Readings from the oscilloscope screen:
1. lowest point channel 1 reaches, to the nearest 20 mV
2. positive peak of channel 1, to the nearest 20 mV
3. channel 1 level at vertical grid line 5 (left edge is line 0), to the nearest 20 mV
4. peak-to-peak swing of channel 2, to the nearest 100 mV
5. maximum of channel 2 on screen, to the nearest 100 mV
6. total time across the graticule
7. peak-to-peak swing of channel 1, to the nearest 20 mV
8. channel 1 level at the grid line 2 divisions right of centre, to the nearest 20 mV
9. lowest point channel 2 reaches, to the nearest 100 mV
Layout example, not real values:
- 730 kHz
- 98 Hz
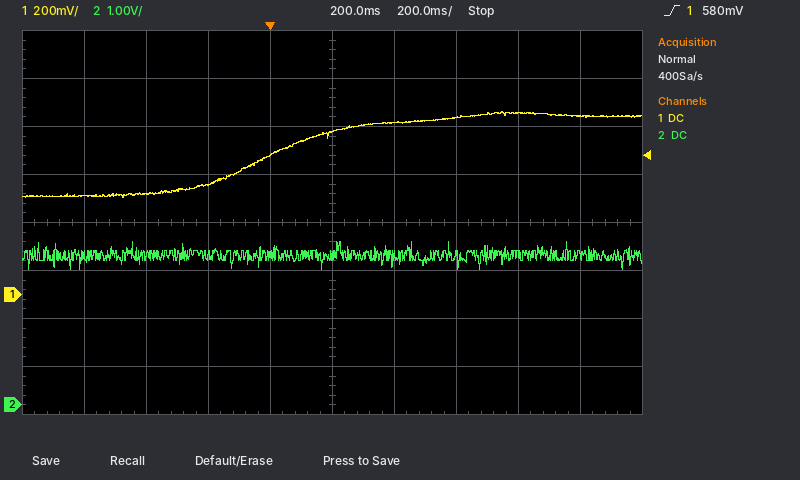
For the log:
- 400 mV
- 760 mV
- 680 mV
- 600 mV
- 3.4 V
- 2 s
- 360 mV
- 740 mV
- 2.8 V
